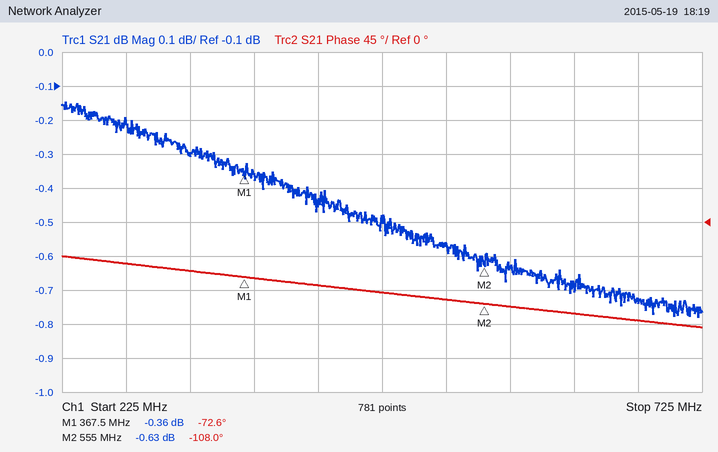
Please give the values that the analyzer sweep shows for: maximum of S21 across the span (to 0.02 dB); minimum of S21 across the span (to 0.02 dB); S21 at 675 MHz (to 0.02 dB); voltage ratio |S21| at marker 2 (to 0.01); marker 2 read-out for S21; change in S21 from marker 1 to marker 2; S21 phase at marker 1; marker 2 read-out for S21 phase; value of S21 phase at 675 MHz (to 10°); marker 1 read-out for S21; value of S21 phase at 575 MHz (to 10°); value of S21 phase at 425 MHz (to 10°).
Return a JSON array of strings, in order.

["-0.14 dB", "-0.78 dB", "-0.74 dB", "0.93", "-0.63 dB", "-0.27 dB", "-72.6°", "-108.0°", "-130°", "-0.36 dB", "-110°", "-80°"]
